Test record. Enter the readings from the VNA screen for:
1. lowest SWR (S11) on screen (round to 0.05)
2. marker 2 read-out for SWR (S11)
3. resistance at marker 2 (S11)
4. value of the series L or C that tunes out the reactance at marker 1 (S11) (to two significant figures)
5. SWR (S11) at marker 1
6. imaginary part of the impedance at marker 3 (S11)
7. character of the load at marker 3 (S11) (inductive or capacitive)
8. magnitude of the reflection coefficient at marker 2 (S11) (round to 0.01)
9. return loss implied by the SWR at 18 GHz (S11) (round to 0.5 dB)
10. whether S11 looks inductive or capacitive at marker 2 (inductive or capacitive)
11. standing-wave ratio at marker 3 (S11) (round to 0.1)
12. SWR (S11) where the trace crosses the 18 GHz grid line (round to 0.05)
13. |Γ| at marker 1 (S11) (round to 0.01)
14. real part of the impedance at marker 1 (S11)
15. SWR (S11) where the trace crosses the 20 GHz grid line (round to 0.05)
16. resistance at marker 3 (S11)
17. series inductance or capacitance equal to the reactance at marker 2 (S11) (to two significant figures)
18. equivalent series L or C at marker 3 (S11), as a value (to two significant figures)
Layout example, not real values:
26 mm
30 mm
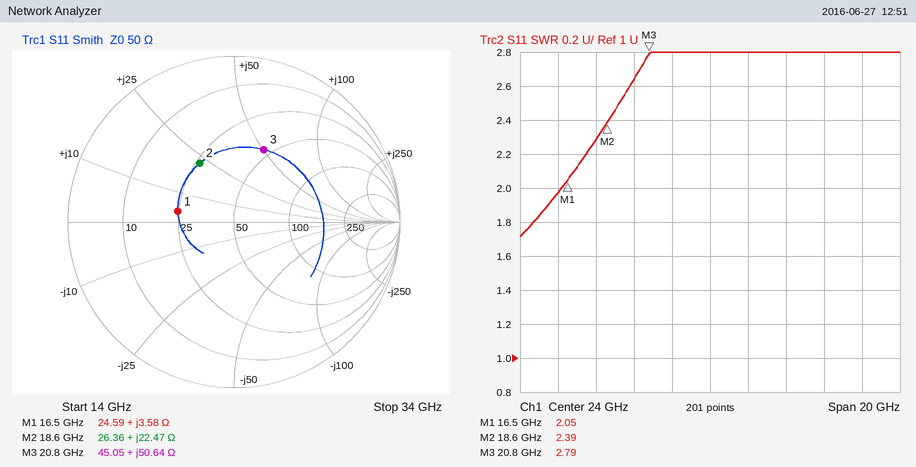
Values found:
1.70
2.39
26.36 Ω
2.7 pF
2.05
+50.64 Ω
inductive
0.41
8.0 dB
inductive
2.8
2.30
0.34
24.59 Ω
2.65
45.05 Ω
190 pH
390 pH
